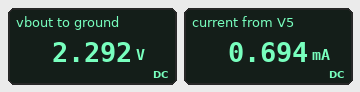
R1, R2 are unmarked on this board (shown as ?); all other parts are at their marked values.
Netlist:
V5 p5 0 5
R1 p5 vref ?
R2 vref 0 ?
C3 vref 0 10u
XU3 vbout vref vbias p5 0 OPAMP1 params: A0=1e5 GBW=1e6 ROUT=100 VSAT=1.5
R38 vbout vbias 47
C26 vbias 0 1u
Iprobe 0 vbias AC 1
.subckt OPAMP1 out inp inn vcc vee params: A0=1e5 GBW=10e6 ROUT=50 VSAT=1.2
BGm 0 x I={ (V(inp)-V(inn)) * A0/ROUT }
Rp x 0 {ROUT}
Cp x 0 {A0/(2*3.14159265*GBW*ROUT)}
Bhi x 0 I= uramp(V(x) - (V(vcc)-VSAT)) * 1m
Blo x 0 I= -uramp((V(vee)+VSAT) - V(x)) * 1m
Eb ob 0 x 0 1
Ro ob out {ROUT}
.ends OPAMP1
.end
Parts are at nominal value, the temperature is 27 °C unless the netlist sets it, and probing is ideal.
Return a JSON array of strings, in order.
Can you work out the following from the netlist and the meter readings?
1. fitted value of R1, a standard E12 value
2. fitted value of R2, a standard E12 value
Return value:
["3.9 kΩ", "3.3 kΩ"]
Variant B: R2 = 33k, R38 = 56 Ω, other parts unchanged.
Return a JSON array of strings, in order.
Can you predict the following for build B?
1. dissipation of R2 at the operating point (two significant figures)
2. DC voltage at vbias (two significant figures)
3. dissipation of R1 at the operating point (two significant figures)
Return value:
["610 µW", "4.5 V", "72 µW"]
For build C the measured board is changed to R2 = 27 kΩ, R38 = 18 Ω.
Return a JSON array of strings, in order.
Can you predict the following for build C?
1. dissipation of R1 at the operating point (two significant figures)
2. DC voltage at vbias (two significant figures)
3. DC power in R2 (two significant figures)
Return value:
["100 µW", "4.4 V", "710 µW"]
